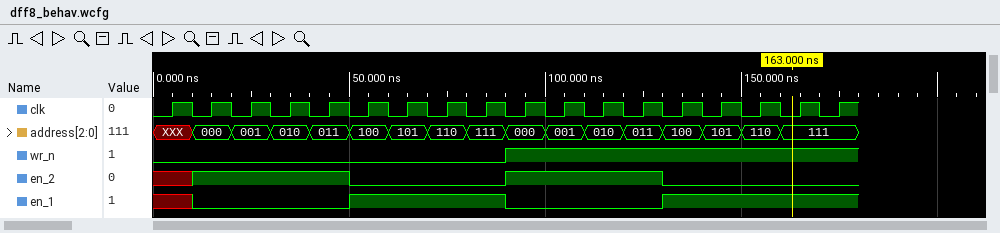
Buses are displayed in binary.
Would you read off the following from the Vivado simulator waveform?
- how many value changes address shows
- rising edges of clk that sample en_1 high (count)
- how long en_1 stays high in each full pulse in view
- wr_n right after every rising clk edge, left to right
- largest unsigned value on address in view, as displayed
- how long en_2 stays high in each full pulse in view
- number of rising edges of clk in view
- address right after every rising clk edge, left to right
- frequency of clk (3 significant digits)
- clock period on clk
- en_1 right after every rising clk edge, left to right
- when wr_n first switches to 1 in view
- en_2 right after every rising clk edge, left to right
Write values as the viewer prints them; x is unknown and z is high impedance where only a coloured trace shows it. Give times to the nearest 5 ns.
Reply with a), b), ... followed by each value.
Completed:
a) 16
b) 9
c) 40 ns
d) 0 0 0 0 0 0 0 0 0 1 1 1 1 1 1 1 1 1
e) 111
f) 40 ns
g) 18
h) XXX, 000, 001, 010, 011, 100, 101, 110, 111, 000, 001, 010, 011, 100, 101, 110, 111, 111
i) 100 MHz
j) 10 ns
k) x 0 0 0 0 1 1 1 1 0 0 0 0 1 1 1 1 1
l) 90 ns
m) x 1 1 1 1 0 0 0 0 1 1 1 1 0 0 0 0 0
